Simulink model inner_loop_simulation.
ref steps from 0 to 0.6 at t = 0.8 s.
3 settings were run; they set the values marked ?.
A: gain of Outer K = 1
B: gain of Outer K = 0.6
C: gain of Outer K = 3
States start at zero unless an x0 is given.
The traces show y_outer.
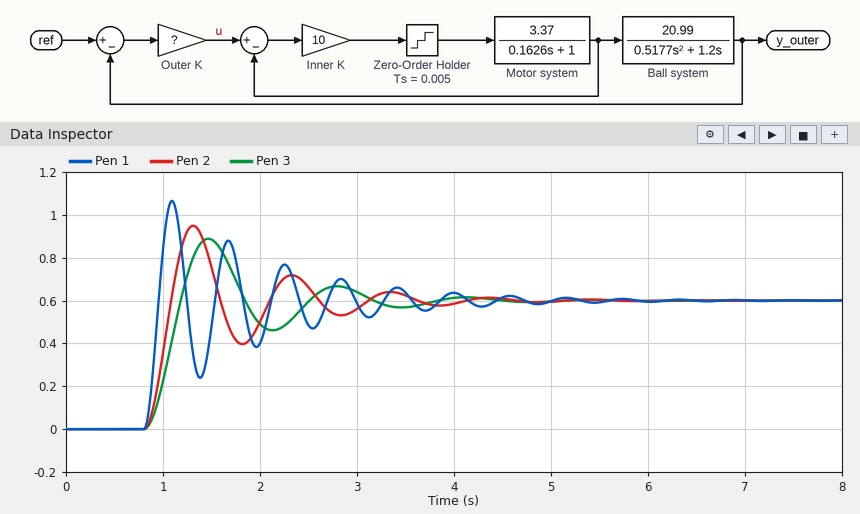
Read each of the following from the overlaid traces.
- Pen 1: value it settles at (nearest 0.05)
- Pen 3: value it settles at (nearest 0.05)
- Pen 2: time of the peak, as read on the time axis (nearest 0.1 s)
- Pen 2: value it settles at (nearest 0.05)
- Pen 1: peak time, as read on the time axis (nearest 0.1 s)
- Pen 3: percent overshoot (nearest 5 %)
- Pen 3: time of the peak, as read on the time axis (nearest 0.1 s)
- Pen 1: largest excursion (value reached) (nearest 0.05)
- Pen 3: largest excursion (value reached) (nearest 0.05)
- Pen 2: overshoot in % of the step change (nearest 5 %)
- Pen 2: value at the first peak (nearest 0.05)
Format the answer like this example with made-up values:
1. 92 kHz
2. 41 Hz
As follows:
1. 0.60
2. 0.60
3. 1.3 s
4. 0.60
5. 1.1 s
6. 50 %
7. 1.5 s
8. 1.05
9. 0.90
10. 60 %
11. 0.95
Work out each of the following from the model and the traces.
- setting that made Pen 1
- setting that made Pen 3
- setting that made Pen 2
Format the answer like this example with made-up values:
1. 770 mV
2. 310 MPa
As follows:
1. C
2. B
3. A
